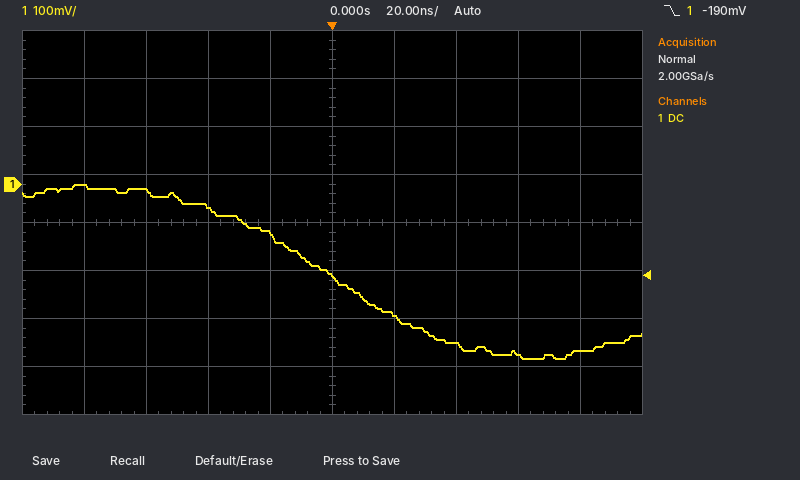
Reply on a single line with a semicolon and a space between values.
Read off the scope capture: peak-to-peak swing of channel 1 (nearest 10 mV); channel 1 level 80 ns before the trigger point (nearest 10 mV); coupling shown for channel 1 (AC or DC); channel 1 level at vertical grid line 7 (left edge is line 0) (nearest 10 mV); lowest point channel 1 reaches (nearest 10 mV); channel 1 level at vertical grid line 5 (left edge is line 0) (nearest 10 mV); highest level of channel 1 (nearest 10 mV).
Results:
360 mV; 0 mV; DC; -330 mV; -360 mV; -190 mV; 0 mV
